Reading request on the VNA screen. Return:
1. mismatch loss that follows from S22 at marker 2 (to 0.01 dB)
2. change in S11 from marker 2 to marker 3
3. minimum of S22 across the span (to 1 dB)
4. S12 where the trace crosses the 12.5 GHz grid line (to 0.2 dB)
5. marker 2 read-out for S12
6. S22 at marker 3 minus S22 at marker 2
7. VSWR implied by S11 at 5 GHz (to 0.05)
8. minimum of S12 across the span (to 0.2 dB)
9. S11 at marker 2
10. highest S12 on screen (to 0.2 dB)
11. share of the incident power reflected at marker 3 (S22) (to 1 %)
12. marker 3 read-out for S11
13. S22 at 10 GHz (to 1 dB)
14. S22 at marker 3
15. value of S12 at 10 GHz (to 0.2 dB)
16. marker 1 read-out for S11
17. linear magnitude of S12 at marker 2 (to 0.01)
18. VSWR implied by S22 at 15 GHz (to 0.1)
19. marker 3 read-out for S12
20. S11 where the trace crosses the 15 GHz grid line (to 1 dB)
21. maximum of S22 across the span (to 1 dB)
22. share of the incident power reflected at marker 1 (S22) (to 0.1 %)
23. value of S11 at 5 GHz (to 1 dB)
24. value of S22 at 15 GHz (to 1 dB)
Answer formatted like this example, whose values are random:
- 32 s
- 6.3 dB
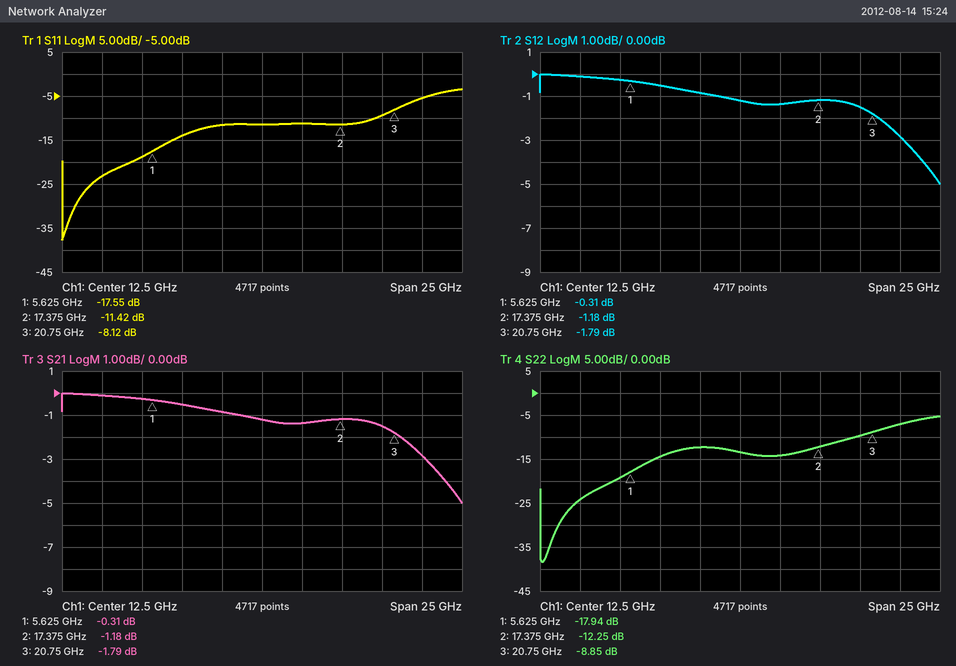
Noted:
- 0.27 dB
- 3.30 dB
- -38 dB
- -1.2 dB
- -1.18 dB
- 3.40 dB
- 1.25
- -5.0 dB
- -11.42 dB
- 0.0 dB
- 13 %
- -8.12 dB
- -12 dB
- -8.85 dB
- -0.8 dB
- -17.55 dB
- 0.87
- 1.5
- -1.79 dB
- -11 dB
- -5 dB
- 1.6 %
- -19 dB
- -14 dB
